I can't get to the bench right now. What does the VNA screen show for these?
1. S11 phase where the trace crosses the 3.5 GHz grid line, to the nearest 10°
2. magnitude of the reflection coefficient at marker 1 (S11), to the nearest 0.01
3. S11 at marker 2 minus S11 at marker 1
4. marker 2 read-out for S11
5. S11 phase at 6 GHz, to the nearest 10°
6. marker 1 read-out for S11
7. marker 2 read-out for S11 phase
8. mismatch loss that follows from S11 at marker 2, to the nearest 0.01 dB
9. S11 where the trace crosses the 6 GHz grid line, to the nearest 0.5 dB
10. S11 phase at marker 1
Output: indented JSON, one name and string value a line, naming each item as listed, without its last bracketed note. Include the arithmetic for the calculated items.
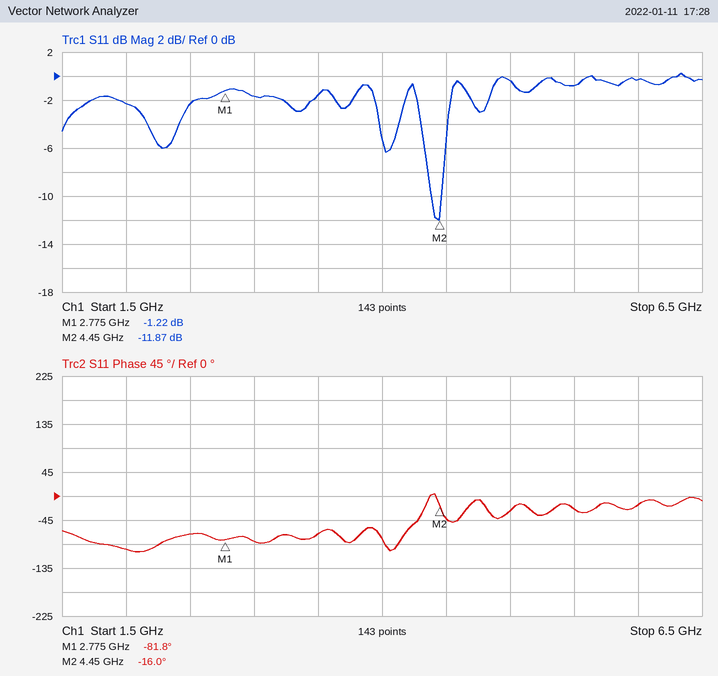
{
  "S11 phase where the trace crosses the 3.5 GHz grid line, to the nearest 10°": "-70°",
  "magnitude of the reflection coefficient at marker 1 (S11), to the nearest 0.01": "10^(-1.22/20) ≈ 0.87",
  "S11 at marker 2 minus S11 at marker 1": "-11.87 − (-1.22) = -10.65 dB",
  "marker 2 read-out for S11": "-11.87 dB",
  "S11 phase at 6 GHz, to the nearest 10°": "-20°",
  "marker 1 read-out for S11": "-1.22 dB",
  "marker 2 read-out for S11 phase": "-16.0°",
  "mismatch loss that follows from S11 at marker 2, to the nearest 0.01 dB": "−10 log10(1 − 10^(-11.87/10)) ≈ 0.29 dB",
  "S11 where the trace crosses the 6 GHz grid line, to the nearest 0.5 dB": "-0.5 dB",
  "S11 phase at marker 1": "-81.8°"
}
